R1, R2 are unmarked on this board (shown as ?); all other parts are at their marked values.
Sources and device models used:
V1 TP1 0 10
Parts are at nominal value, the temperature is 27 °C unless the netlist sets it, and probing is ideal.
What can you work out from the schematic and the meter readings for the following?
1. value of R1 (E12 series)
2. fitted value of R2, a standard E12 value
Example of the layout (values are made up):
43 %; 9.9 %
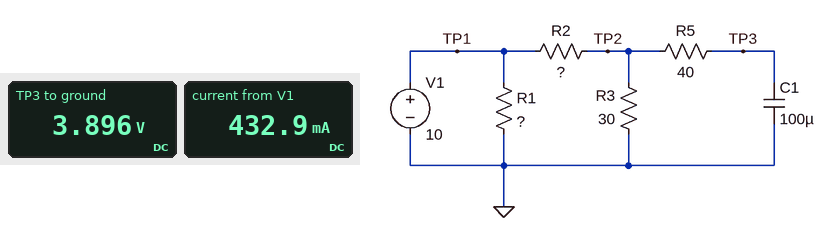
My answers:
33 Ω; 47 Ω
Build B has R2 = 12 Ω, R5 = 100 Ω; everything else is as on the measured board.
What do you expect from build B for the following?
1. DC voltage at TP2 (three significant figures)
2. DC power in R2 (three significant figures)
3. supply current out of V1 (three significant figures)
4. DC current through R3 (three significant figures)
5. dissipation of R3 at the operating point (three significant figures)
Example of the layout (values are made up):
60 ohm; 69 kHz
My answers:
7.14 V; 680 mW; 541 mA; 238 mA; 1.70 W
